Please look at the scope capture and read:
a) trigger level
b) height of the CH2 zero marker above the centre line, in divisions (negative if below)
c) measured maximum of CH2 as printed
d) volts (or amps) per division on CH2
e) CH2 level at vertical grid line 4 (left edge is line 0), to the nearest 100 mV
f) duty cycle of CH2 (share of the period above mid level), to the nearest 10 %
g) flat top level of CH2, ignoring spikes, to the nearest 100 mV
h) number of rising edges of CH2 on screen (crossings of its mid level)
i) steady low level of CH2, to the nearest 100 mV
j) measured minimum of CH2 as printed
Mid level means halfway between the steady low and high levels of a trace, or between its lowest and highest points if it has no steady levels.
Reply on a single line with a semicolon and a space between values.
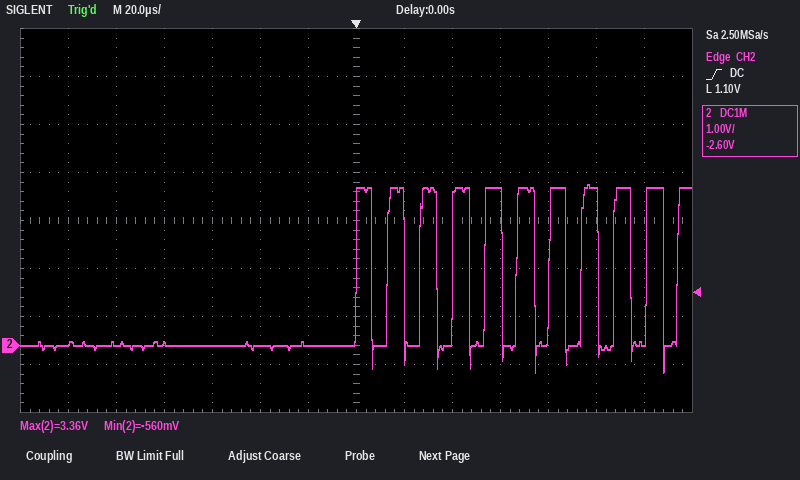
1.10 V; -2.6 div; 3.36 V; 1 V; 0.0 V; 50 %; 3.3 V; 11; 0.0 V; -560 mV
